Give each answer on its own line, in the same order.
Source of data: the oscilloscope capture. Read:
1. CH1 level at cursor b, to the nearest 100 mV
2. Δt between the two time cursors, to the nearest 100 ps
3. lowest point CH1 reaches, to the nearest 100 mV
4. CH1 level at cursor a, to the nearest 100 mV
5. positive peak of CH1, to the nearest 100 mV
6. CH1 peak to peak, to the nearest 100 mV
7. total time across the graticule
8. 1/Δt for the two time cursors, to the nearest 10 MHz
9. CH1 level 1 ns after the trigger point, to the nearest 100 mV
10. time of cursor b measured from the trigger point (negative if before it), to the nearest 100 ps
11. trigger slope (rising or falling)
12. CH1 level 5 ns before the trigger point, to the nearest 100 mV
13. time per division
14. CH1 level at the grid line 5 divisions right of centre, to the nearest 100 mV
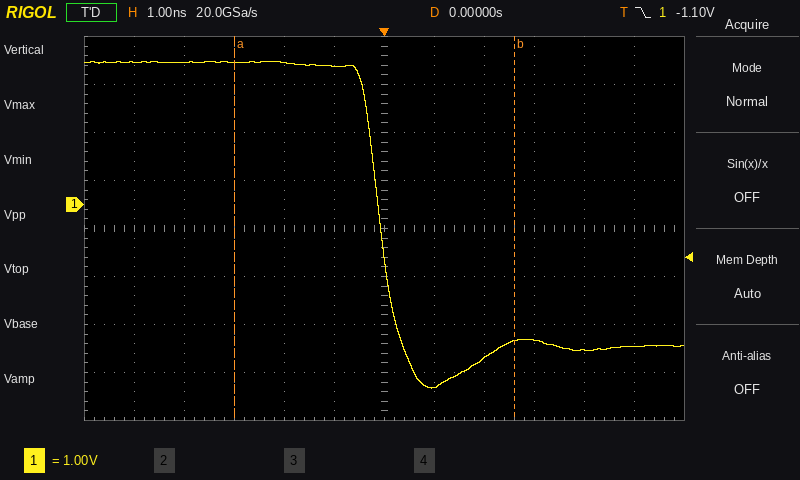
-2.8 V
5.6 ns
-3.8 V
3.0 V
3.0 V
6.8 V
12 ns
180 MHz
-3.8 V
+2.6 ns
falling
3.0 V
1 ns
-3.0 V
